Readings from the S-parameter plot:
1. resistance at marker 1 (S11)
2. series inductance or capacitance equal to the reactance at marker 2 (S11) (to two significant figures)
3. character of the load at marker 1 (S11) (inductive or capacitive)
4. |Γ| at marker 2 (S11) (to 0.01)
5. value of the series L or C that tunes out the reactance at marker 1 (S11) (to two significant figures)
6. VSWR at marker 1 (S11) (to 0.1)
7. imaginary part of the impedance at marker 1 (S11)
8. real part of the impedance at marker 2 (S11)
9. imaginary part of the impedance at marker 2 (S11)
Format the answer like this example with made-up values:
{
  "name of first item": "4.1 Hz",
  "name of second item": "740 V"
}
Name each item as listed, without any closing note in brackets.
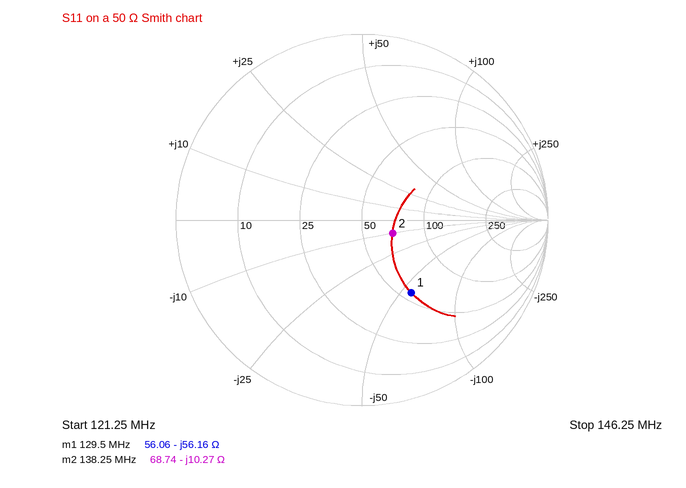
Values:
{
  "resistance at marker 1": "56.06 Ω",
  "series inductance or capacitance equal to the reactance at marker 2 (S11)": "110 pF",
  "character of the load at marker 1 (S11)": "capacitive",
  "|Γ| at marker 2 (S11)": "0.18",
  "value of the series L or C that tunes out the reactance at marker 1 (S11)": "69 nH",
  "VSWR at marker 1 (S11)": "2.8",
  "imaginary part of the impedance at marker 1": "-56.16 Ω",
  "real part of the impedance at marker 2": "68.74 Ω",
  "imaginary part of the impedance at marker 2": "-10.27 Ω"
}
